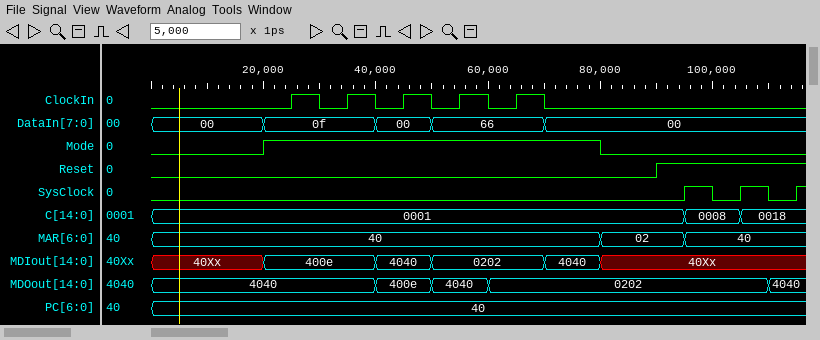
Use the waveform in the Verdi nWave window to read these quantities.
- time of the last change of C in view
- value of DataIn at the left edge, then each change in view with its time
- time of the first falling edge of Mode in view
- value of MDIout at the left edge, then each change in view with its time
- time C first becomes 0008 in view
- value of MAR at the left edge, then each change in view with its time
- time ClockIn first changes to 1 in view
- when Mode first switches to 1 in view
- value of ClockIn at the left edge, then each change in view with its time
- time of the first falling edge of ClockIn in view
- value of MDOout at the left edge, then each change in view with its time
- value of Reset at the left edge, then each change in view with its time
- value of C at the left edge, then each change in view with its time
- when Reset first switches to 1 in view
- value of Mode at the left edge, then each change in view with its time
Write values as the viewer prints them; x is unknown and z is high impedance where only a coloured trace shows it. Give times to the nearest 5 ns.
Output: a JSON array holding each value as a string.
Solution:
["105 ns", "00, 0f at 20 ns, 00 at 40 ns, 66 at 50 ns, 00 at 70 ns", "80 ns", "40Xx, 400e at 20 ns, 4040 at 40 ns, 0202 at 50 ns, 4040 at 70 ns, 40Xx at 80 ns", "95 ns", "40, 02 at 80 ns, 40 at 95 ns", "25 ns", "20 ns", "0, 1 at 25 ns, 0 at 30 ns, 1 at 35 ns, 0 at 40 ns, 1 at 45 ns, 0 at 50 ns, 1 at 55 ns, 0 at 60 ns, 1 at 65 ns, 0 at 70 ns", "30 ns", "4040, 400e at 40 ns, 4040 at 50 ns, 0202 at 60 ns, 4040 at 110 ns", "0, 1 at 90 ns", "0001, 0008 at 95 ns, 0018 at 105 ns", "90 ns", "0, 1 at 20 ns, 0 at 80 ns"]
